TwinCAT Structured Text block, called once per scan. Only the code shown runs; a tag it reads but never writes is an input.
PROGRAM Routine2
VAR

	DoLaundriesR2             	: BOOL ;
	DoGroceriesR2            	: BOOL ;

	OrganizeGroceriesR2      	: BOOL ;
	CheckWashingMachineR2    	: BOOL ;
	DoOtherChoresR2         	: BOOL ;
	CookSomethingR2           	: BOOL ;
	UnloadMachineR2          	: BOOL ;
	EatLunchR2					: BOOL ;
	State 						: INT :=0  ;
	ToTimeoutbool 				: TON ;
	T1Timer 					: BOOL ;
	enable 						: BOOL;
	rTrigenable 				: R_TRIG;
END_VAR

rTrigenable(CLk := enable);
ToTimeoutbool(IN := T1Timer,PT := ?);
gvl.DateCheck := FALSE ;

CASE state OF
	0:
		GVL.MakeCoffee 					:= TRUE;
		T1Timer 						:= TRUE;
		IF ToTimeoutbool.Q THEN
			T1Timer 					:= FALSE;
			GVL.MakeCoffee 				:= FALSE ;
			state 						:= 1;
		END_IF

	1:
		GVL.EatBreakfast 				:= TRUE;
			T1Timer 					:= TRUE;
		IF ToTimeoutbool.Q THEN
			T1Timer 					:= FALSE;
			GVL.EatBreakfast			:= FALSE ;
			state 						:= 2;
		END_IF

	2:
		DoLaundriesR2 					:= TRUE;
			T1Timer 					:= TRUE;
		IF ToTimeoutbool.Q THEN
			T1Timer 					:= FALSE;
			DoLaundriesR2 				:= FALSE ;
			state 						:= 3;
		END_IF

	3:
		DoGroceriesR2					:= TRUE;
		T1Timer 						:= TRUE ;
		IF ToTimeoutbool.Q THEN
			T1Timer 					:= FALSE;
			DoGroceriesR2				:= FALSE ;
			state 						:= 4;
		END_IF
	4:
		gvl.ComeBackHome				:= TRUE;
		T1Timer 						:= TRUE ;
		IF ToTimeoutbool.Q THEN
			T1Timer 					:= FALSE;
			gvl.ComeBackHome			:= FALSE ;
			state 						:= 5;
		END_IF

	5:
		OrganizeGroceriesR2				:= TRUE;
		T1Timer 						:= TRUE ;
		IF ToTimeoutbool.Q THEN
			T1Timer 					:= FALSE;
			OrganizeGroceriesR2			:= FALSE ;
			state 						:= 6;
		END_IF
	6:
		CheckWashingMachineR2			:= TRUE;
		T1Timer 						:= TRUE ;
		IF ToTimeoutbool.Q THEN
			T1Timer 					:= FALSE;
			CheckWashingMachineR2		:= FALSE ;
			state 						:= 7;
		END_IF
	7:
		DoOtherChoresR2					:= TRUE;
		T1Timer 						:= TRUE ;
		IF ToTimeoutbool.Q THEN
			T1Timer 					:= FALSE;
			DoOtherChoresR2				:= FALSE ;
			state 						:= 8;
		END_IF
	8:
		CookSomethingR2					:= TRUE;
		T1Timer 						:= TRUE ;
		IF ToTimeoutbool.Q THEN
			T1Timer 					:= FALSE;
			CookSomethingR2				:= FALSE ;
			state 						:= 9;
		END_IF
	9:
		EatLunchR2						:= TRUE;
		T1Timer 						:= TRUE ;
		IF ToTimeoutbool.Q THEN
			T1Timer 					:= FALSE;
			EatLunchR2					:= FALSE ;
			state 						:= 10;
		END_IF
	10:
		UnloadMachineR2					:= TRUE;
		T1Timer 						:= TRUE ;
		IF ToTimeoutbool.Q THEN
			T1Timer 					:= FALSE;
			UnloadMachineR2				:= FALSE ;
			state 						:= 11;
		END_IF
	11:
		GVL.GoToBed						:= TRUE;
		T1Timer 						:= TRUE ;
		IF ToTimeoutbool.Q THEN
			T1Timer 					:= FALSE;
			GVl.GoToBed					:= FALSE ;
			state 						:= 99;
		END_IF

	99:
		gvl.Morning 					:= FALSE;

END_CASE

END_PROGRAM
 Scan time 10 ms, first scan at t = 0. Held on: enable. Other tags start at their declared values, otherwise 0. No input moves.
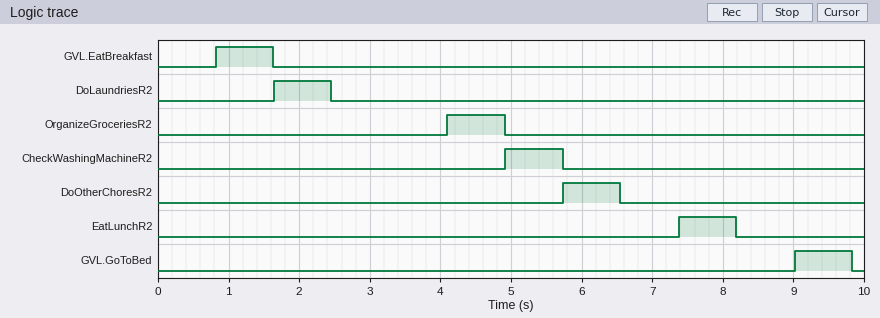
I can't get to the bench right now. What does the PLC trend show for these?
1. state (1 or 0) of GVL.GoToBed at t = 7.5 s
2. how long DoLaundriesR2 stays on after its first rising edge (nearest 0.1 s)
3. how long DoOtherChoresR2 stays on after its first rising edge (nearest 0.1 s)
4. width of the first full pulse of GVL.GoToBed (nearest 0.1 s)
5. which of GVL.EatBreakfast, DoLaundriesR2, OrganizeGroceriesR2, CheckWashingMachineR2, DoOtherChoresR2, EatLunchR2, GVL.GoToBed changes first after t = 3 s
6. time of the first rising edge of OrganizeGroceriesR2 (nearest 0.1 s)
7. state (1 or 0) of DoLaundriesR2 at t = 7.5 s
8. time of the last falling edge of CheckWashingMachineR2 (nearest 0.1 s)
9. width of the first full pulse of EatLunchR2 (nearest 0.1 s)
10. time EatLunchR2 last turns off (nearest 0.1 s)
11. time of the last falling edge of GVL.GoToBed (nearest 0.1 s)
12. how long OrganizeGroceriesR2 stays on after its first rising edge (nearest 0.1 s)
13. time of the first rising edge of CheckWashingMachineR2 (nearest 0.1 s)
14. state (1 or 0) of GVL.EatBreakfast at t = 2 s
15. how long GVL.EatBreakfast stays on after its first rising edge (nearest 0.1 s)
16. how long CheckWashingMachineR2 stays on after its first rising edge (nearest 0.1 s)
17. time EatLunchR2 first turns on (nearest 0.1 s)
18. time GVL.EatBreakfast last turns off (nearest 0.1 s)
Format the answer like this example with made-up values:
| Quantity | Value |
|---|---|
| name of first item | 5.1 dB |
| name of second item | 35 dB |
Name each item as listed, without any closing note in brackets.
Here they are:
| Quantity | Value |
|---|---|
| state (1 or 0) of GVL.GoToBed at t = 7.5 s | 0 |
| how long DoLaundriesR2 stays on after its first rising edge | 0.8 s |
| how long DoOtherChoresR2 stays on after its first rising edge | 0.8 s |
| width of the first full pulse of GVL.GoToBed | 0.8 s |
| which of GVL.EatBreakfast, DoLaundriesR2, OrganizeGroceriesR2, CheckWashingMachineR2, DoOtherChoresR2, EatLunchR2, GVL.GoToBed changes first after t = 3 s | OrganizeGroceriesR2 |
| time of the first rising edge of OrganizeGroceriesR2 | 4.1 s |
| state (1 or 0) of DoLaundriesR2 at t = 7.5 s | 0 |
| time of the last falling edge of CheckWashingMachineR2 | 5.7 s |
| width of the first full pulse of EatLunchR2 | 0.8 s |
| time EatLunchR2 last turns off | 8.2 s |
| time of the last falling edge of GVL.GoToBed | 9.8 s |
| how long OrganizeGroceriesR2 stays on after its first rising edge | 0.8 s |
| time of the first rising edge of CheckWashingMachineR2 | 4.9 s |
| state (1 or 0) of GVL.EatBreakfast at t = 2 s | 0 |
| how long GVL.EatBreakfast stays on after its first rising edge | 0.8 s |
| how long CheckWashingMachineR2 stays on after its first rising edge | 0.8 s |
| time EatLunchR2 first turns on | 7.4 s |
| time GVL.EatBreakfast last turns off | 1.6 s |
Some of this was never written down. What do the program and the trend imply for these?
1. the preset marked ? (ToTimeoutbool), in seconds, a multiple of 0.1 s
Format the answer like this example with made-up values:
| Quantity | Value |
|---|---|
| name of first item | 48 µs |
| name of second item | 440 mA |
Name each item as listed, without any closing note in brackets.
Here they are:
| Quantity | Value |
|---|---|
| the preset marked ? (ToTimeoutbool), in seconds, a multiple of 0.1 s | 0.8 s |
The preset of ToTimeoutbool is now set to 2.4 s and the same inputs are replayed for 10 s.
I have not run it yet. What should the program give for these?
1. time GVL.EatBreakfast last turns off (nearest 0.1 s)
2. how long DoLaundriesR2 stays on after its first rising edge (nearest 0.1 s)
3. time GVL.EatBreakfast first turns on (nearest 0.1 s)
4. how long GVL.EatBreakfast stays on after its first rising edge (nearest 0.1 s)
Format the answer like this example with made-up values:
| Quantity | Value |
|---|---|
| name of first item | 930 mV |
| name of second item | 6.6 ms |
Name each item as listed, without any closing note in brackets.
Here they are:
| Quantity | Value |
|---|---|
| time GVL.EatBreakfast last turns off | 4.8 s |
| how long DoLaundriesR2 stays on after its first rising edge | 2.4 s |
| time GVL.EatBreakfast first turns on | 2.4 s |
| how long GVL.EatBreakfast stays on after its first rising edge | 2.4 s |
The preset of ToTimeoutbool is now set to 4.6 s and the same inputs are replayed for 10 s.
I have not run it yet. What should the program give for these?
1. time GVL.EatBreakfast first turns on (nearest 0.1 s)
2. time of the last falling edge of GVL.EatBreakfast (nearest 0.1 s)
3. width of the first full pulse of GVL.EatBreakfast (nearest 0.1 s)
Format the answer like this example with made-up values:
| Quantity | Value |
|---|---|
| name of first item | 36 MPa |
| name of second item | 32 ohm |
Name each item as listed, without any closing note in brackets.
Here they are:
| Quantity | Value |
|---|---|
| time GVL.EatBreakfast first turns on | 4.6 s |
| time of the last falling edge of GVL.EatBreakfast | 9.2 s |
| width of the first full pulse of GVL.EatBreakfast | 4.6 s |
